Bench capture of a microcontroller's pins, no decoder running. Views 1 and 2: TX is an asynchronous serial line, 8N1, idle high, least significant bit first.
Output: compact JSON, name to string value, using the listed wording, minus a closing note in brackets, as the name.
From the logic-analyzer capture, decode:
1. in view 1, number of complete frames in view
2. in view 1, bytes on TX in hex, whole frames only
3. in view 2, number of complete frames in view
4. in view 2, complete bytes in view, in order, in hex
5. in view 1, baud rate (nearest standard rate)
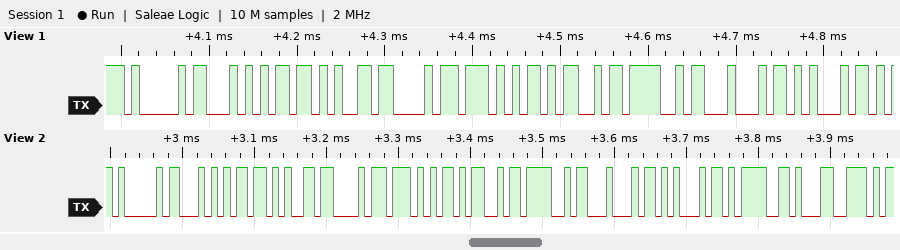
{"in view 1, number of complete frames in view": "9", "in view 1, bytes on TX in hex, whole frames only": "41 54 2B 43 57 4D 4F 44 45", "in view 2, number of complete frames in view": "11", "in view 2, complete bytes in view, in order, in hex": "0x41 0x54 0x2B 0x43 0x57 0x4D 0x4F 0x44 0x45 0x3D 0x31", "in view 1, baud rate": "115200 baud"}
